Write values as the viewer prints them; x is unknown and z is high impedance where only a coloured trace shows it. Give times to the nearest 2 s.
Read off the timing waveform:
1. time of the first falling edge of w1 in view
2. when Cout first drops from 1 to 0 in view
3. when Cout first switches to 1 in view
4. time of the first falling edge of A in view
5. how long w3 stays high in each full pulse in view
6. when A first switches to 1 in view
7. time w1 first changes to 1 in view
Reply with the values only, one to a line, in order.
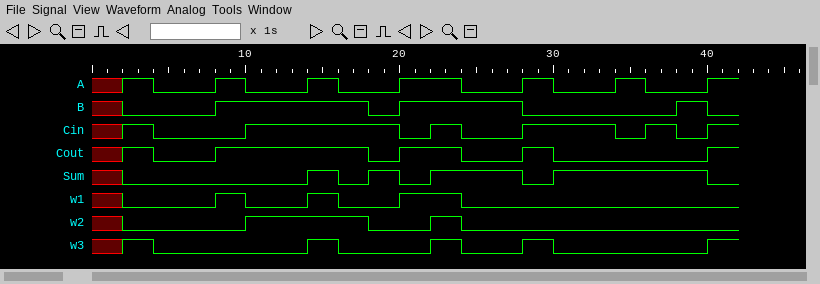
10 s
4 s
2 s
4 s
2 s, 2 s, 2 s
2 s
8 s
